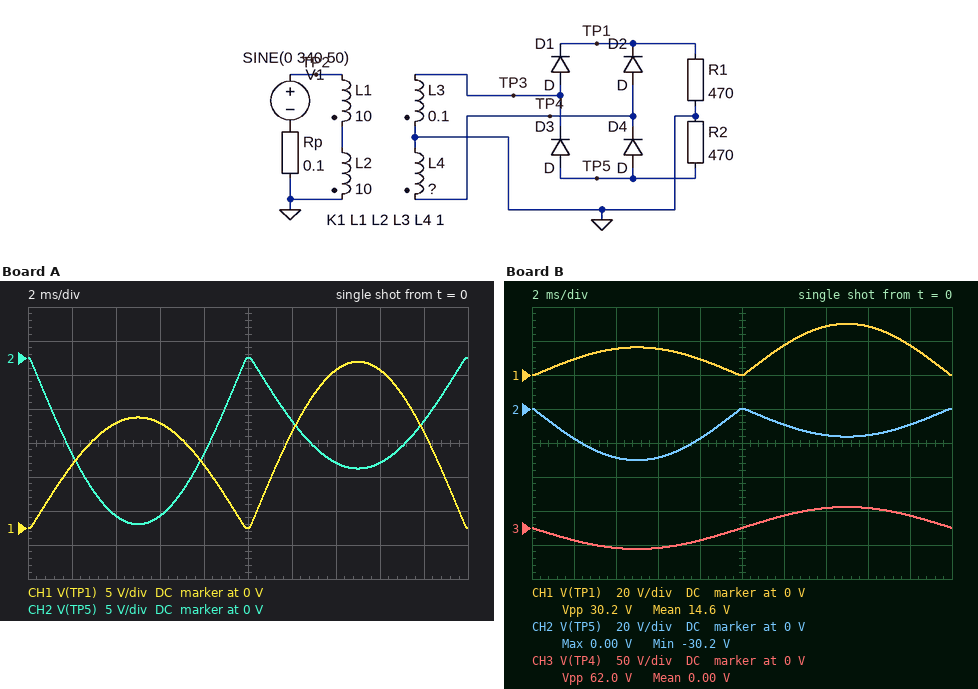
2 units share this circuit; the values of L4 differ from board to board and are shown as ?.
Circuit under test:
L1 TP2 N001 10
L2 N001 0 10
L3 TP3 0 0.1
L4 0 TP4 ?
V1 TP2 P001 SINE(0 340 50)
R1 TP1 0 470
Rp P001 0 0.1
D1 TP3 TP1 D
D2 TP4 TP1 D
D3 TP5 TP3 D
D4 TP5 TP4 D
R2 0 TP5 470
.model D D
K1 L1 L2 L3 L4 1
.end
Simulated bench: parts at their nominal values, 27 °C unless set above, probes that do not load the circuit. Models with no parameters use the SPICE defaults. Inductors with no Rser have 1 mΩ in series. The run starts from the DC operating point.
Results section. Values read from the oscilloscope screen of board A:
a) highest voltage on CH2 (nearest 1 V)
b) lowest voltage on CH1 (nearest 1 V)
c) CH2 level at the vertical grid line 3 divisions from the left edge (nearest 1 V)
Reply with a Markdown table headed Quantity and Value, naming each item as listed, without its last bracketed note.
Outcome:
| Quantity | Value |
|---|---|
| highest voltage on CH2 | 0 V |
| lowest voltage on CH1 | 0 V |
| CH2 level at the vertical grid line 3 divisions from the left edge | -23 V |
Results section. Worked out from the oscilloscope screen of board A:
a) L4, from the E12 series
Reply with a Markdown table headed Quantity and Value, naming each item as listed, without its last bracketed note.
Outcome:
| Quantity | Value |
|---|---|
| L4, from the E12 series | 220 mH |
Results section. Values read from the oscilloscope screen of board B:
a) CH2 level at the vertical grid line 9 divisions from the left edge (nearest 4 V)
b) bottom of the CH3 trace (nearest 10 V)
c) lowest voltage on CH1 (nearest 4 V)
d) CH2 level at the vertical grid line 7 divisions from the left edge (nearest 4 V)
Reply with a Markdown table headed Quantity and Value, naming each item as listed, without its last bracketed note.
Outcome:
| Quantity | Value |
|---|---|
| CH2 level at the vertical grid line 9 divisions from the left edge | -8 V |
| bottom of the CH3 trace | -30 V |
| lowest voltage on CH1 | 0 V |
| CH2 level at the vertical grid line 7 divisions from the left edge | -16 V |
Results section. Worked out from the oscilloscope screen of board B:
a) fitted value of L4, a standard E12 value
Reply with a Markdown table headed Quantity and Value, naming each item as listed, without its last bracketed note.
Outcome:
| Quantity | Value |
|---|---|
| fitted value of L4, a standard E12 value | 330 mH |
